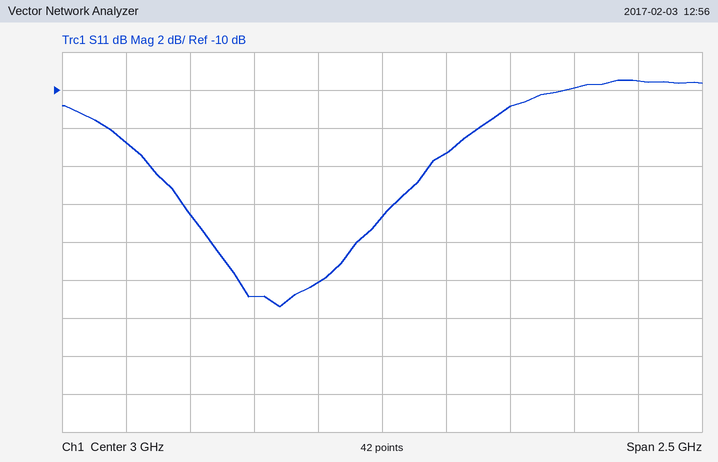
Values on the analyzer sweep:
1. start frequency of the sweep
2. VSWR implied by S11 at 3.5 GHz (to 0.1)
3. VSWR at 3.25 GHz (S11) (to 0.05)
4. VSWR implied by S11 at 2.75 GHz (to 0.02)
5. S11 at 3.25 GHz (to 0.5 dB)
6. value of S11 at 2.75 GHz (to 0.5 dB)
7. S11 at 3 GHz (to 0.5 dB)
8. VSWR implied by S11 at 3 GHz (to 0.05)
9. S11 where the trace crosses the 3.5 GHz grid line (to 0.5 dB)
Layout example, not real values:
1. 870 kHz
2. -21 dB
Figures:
1. 1.75 GHz
2. 1.8
3. 1.55
4. 1.22
5. -13.5 dB
6. -20.0 dB
7. -16.5 dB
8. 1.35
9. -11.0 dB
